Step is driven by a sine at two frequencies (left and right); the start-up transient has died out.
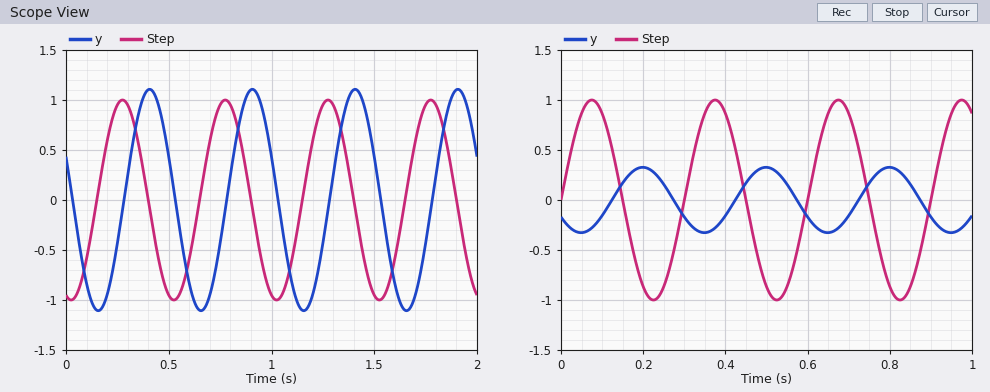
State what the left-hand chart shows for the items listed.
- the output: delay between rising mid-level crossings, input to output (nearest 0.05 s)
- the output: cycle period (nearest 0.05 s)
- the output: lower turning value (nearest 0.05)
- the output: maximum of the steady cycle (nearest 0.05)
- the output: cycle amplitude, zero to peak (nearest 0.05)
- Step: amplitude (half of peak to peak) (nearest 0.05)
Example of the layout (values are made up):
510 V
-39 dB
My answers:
0.15 s
0.50 s
-1.10
1.10
1.10
1.00
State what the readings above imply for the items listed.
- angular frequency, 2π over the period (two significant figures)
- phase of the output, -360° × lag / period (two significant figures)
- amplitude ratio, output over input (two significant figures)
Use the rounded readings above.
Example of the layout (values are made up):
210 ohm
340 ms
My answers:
13 rad/s
-110°
1.1
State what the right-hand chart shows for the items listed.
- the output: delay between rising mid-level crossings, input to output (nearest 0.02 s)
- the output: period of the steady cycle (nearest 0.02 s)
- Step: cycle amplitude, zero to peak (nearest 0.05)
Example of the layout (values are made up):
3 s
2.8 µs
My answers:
0.12 s
0.30 s
1.00
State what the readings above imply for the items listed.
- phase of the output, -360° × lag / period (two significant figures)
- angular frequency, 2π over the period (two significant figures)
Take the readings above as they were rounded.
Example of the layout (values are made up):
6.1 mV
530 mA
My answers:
-140°
21 rad/s
